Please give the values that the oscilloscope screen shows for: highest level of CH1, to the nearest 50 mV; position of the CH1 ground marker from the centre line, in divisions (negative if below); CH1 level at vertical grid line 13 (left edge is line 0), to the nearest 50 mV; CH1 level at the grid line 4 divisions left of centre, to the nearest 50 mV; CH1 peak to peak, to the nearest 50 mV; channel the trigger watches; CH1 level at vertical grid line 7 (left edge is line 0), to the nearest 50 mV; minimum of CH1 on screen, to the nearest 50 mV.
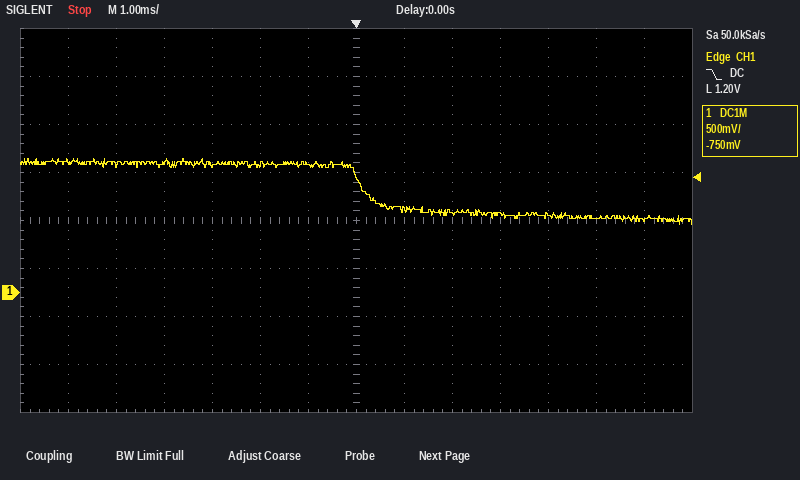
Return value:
1.40 V
-1.5 div
750 mV
1.35 V
700 mV
CH1
1.20 V
700 mV
